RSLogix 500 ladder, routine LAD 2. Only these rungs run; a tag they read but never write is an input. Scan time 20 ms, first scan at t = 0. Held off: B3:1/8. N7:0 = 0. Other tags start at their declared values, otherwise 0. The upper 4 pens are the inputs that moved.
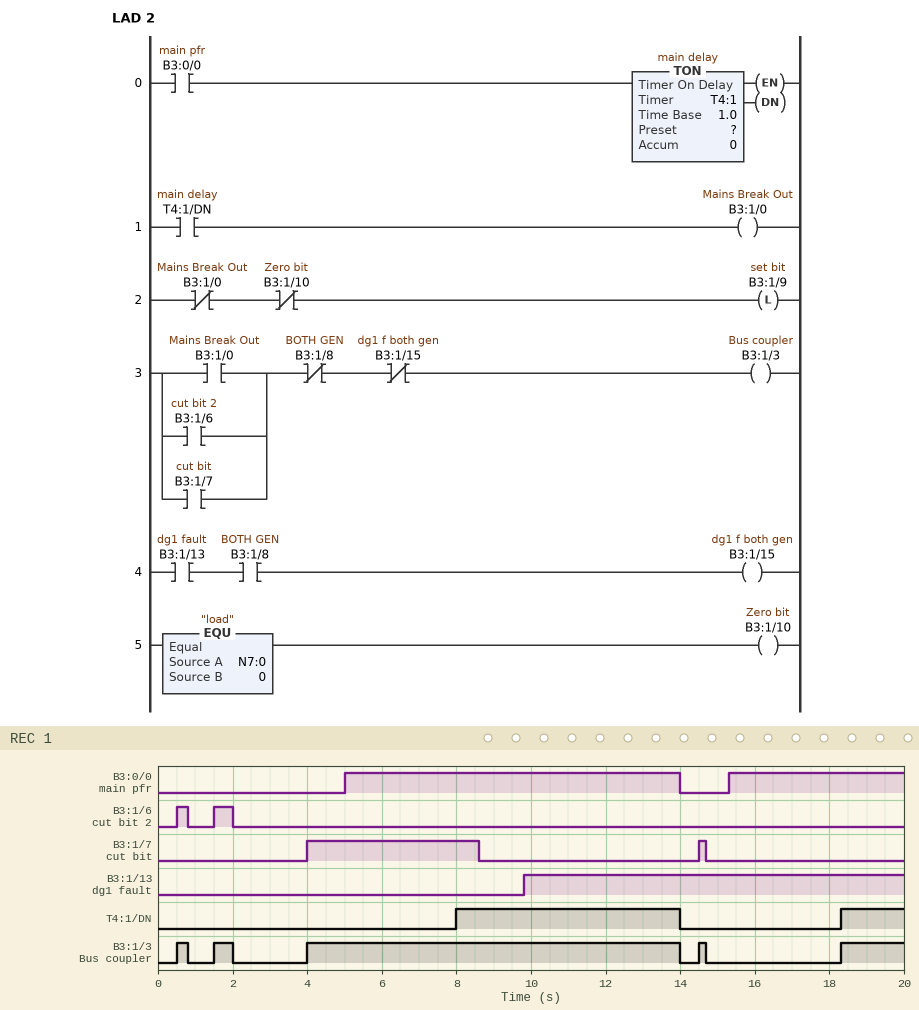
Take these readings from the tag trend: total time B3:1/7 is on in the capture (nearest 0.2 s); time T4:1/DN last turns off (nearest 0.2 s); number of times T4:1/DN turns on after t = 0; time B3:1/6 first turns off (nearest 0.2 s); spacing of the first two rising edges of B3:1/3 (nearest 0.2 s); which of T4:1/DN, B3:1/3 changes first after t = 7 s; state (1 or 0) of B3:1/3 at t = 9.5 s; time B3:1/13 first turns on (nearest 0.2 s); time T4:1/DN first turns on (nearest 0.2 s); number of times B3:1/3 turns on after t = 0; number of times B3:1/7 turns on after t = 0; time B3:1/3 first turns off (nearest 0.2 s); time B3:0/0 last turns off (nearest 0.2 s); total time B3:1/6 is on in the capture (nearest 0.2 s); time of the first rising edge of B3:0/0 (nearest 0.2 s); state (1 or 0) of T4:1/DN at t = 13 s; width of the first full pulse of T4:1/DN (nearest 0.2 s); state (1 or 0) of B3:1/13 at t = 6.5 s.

4.8 s
14.0 s
2
0.8 s
1.0 s
T4:1/DN
1
9.8 s
8.0 s
5
2
0.8 s
14.0 s
0.8 s
5.0 s
1
6.0 s
0
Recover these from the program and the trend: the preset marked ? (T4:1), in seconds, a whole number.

3 s
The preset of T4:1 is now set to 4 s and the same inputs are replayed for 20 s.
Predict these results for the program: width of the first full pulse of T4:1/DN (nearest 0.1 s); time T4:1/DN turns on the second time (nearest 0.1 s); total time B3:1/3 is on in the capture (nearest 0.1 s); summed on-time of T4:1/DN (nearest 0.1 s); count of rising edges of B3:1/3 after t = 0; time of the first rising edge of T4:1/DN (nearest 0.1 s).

5.0 s
19.3 s
11.3 s
5.7 s
6
9.0 s
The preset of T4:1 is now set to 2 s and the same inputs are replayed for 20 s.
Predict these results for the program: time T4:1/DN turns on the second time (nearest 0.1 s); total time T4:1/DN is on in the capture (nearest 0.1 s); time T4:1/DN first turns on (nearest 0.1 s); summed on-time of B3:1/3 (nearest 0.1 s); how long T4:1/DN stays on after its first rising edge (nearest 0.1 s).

17.3 s
9.7 s
7.0 s
13.7 s
7.0 s
